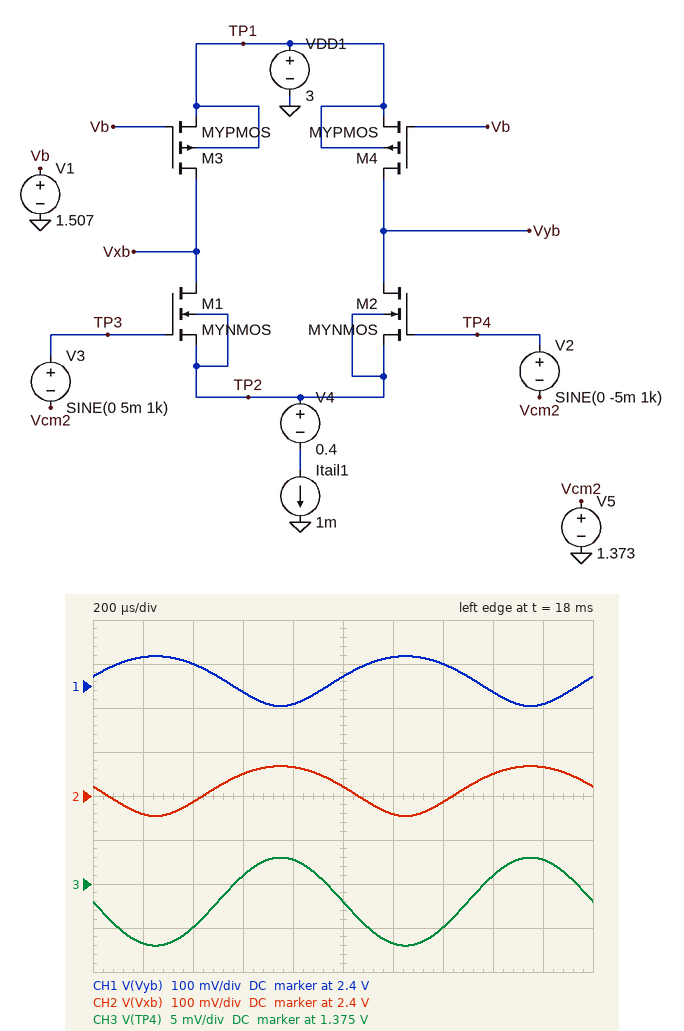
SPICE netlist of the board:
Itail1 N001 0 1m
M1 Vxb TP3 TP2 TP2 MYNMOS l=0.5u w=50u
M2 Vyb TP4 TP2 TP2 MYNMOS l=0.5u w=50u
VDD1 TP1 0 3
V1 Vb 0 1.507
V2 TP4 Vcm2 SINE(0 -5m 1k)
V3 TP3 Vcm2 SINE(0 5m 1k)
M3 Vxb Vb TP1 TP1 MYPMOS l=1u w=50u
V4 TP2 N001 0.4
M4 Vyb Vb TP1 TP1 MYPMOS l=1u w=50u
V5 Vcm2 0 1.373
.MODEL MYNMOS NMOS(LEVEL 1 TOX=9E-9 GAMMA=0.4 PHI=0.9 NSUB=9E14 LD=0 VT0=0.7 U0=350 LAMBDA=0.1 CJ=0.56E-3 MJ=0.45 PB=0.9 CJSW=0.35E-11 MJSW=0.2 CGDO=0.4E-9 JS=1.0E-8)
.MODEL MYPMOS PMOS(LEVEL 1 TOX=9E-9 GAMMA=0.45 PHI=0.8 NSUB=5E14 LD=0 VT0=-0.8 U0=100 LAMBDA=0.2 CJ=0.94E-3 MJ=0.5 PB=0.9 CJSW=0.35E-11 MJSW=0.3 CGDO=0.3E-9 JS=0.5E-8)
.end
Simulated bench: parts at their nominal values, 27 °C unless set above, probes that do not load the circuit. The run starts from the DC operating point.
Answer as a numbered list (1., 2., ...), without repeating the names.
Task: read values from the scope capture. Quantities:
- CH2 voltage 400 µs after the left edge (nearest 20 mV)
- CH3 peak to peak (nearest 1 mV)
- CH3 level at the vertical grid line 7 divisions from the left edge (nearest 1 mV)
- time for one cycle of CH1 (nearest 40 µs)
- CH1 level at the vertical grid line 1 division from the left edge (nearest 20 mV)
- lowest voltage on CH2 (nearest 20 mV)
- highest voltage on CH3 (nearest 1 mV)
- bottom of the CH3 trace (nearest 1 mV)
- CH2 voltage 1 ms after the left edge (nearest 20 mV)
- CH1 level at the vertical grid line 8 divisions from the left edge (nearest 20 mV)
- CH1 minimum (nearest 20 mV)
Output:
1. 2.38 V
2. 10 mV
3. 1.370 V
4. 1.00 ms
5. 2.46 V
6. 2.36 V
7. 1.378 V
8. 1.368 V
9. 2.42 V
10. 2.38 V
11. 2.36 V
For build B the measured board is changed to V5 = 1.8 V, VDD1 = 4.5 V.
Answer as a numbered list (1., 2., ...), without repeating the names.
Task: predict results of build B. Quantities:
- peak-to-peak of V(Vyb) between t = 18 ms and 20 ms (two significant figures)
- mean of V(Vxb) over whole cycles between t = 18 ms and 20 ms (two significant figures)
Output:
1. 10 mV
2. 4.4 V
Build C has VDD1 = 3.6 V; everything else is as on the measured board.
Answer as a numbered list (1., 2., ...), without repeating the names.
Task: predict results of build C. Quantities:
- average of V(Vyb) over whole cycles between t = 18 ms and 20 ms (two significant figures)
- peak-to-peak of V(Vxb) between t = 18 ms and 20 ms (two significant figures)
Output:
1. 3.4 V
2. 18 mV
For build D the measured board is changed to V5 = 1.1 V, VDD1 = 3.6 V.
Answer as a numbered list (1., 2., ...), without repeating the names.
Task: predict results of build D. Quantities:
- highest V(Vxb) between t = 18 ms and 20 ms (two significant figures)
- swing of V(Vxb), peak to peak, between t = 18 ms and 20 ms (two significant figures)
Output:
1. 3.4 V
2. 18 mV
